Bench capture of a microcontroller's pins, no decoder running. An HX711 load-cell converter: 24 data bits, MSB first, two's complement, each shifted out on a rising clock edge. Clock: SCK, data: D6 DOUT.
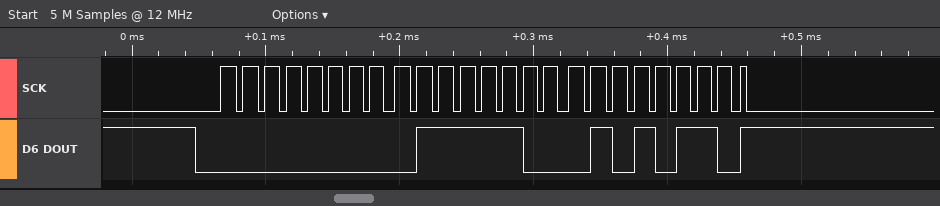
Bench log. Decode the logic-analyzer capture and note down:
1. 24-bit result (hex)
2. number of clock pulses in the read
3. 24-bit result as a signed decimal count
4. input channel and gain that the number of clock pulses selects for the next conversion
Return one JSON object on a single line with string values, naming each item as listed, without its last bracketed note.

{"24-bit result": "0x007C56", "number of clock pulses in the read": "25", "24-bit result as a signed decimal count": "31830", "input channel and gain that the number of clock pulses selects for the next conversion": "channel A, gain 128"}
